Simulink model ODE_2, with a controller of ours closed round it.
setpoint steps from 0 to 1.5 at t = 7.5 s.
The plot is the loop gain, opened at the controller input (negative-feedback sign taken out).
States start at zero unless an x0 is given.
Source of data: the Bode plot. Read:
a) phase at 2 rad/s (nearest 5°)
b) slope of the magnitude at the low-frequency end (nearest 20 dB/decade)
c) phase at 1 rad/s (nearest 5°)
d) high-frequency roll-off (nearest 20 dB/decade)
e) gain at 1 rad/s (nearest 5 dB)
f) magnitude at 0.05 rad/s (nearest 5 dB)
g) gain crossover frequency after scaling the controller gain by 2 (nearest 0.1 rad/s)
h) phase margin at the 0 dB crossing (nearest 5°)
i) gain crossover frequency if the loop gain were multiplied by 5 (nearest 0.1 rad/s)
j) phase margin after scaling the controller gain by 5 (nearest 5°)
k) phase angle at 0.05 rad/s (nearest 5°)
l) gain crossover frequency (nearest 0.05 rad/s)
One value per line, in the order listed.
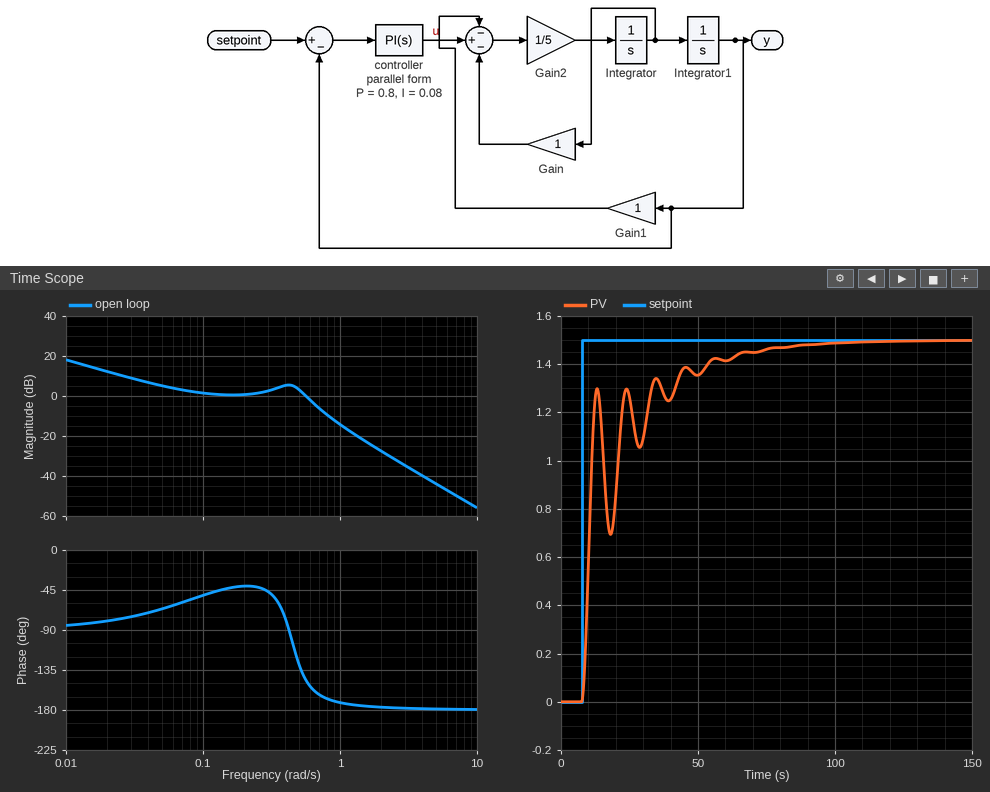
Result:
-175°
-20 dB/decade
-170°
-40 dB/decade
-15 dB
5 dB
0.7 rad/s
35°
1.0 rad/s
10°
-65°
0.55 rad/s
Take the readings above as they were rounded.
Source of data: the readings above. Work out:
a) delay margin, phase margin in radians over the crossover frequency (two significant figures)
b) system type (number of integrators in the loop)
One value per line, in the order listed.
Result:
1.1 s
1
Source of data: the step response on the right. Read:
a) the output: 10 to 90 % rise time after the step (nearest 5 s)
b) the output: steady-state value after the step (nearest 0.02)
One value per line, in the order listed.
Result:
35 s
1.50
